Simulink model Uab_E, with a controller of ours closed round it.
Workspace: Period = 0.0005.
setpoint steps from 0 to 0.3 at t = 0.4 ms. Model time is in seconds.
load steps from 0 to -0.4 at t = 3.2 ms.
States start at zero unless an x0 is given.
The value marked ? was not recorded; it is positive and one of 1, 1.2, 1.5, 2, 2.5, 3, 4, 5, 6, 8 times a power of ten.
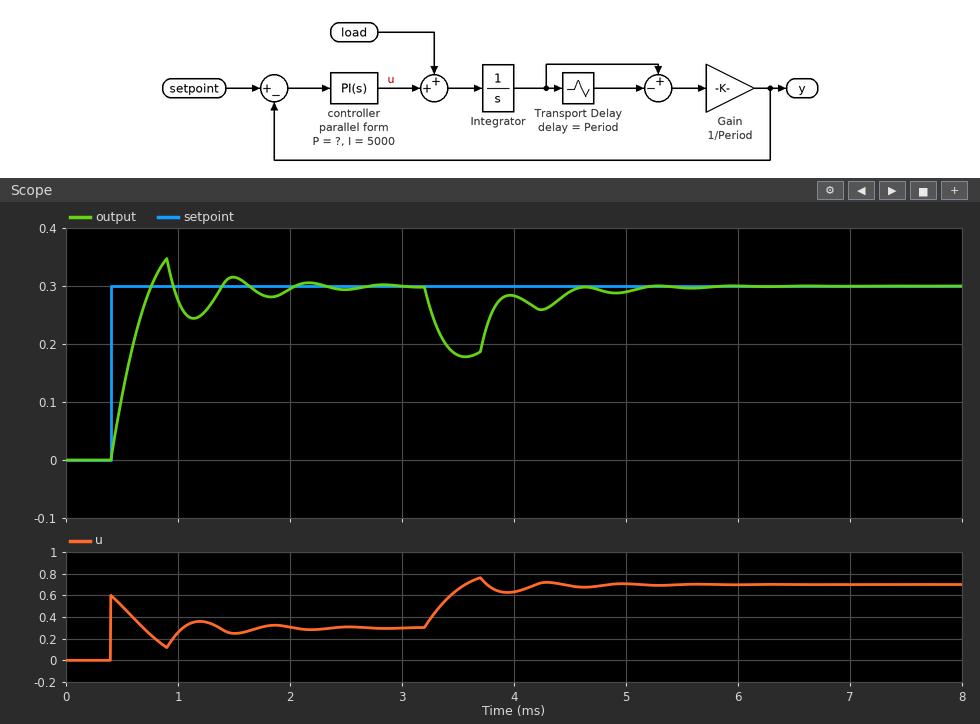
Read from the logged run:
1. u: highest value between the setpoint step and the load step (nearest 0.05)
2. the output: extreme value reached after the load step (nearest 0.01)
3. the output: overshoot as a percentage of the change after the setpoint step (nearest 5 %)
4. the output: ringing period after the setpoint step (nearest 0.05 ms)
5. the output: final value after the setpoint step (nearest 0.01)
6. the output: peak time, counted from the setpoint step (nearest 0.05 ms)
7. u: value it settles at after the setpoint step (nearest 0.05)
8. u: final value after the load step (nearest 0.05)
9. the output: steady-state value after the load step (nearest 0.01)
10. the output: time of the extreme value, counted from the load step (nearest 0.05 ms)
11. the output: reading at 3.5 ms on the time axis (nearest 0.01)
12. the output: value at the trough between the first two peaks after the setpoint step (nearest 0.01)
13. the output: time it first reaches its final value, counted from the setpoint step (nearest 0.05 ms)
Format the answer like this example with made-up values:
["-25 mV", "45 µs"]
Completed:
["0.60", "0.18", "15 %", "0.60 ms", "0.30", "0.50 ms", "0.30", "0.70", "0.30", "0.35 ms", "0.18", "0.24", "0.35 ms"]
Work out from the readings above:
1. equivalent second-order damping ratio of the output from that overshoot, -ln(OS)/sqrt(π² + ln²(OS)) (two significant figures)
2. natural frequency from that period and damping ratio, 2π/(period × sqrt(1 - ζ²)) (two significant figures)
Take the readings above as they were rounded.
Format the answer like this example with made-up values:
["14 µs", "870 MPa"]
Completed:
["0.52", "12 rad/ms"]
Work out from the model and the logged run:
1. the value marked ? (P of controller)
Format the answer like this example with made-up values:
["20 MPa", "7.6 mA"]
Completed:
["2"]
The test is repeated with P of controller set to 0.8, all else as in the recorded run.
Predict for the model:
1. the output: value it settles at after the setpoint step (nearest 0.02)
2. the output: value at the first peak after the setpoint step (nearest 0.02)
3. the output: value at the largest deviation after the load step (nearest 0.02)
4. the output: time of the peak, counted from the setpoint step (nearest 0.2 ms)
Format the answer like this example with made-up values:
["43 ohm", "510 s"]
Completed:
["0.30", "0.34", "0.12", "0.6 ms"]
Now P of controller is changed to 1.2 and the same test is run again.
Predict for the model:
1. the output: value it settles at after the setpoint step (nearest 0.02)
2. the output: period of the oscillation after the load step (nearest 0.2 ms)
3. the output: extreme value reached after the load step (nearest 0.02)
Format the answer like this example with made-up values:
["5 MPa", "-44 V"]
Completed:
["0.30", "0.8 ms", "0.14"]
